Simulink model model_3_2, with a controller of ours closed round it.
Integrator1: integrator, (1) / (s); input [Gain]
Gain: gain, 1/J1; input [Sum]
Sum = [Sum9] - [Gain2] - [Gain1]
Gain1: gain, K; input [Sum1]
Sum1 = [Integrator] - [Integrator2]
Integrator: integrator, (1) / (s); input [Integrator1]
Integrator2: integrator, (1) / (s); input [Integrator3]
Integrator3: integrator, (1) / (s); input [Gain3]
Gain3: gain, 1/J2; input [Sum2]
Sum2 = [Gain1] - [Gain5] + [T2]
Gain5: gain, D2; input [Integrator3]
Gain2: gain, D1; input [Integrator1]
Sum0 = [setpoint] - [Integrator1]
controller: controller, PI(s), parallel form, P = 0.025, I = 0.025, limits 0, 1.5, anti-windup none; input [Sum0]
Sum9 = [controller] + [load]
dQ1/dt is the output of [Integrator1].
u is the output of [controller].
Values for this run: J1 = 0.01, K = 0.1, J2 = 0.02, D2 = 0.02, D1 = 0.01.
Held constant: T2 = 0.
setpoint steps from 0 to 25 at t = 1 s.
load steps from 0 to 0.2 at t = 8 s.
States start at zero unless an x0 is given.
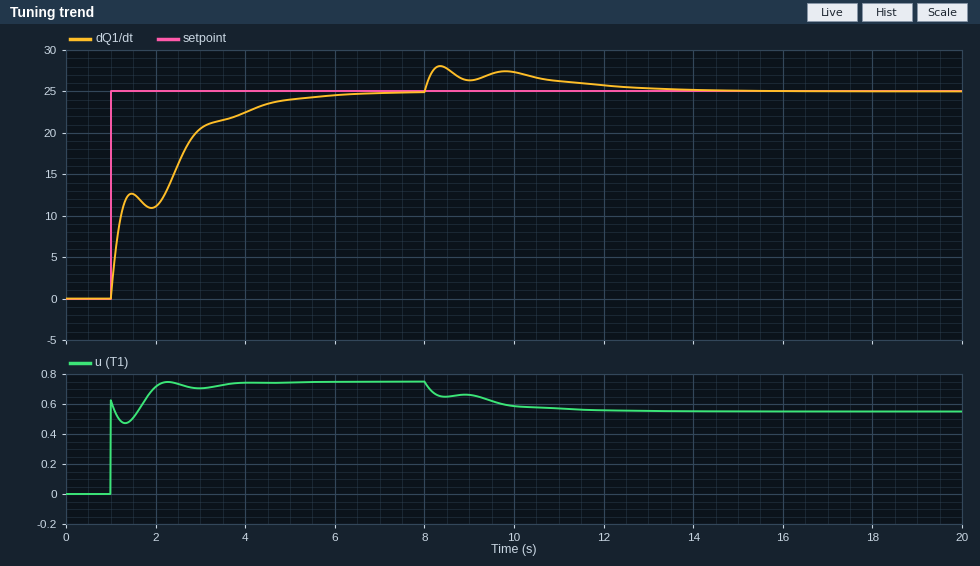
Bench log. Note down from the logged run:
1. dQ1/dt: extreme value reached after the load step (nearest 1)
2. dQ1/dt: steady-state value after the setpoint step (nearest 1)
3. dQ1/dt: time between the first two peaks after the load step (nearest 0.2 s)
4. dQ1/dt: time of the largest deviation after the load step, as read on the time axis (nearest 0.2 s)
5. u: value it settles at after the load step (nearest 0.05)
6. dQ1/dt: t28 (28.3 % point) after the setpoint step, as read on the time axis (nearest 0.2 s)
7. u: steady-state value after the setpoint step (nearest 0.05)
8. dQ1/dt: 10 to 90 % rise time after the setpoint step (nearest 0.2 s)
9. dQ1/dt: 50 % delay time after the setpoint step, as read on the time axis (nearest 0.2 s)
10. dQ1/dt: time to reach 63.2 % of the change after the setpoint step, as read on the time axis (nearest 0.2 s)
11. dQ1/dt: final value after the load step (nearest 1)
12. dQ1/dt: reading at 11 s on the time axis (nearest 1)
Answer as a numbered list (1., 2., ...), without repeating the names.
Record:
1. 28
2. 25
3. 1.4 s
4. 8.4 s
5. 0.55
6. 1.2 s
7. 0.75
8. 3.0 s
9. 1.4 s
10. 2.4 s
11. 25
12. 26
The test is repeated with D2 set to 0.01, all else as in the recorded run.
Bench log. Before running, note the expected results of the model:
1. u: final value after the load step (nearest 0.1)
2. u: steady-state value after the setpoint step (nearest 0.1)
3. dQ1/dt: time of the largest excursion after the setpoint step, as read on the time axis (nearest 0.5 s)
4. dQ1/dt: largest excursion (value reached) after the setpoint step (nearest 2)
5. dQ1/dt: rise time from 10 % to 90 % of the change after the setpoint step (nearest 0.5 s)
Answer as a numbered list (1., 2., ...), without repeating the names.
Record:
1. 0.3
2. 0.5
3. 5.0 s
4. 26
5. 2.0 s
